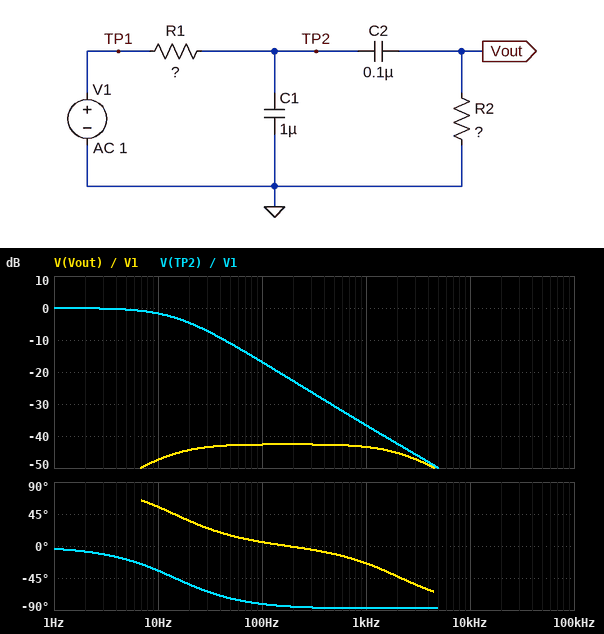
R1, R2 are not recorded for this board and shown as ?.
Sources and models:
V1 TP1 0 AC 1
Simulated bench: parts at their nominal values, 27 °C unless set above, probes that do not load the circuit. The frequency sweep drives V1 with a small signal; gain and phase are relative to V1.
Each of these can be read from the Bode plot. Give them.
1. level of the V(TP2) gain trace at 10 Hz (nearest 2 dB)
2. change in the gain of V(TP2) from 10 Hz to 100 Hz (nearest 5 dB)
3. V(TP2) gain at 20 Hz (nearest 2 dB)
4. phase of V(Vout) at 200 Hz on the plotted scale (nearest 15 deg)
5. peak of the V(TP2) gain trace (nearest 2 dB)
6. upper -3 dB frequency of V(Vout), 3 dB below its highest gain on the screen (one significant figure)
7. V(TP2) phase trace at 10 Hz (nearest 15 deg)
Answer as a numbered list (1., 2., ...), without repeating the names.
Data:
1. -2 dB
2. -15 dB
3. -4 dB
4. 0 deg
5. 0 dB
6. 2 kHz
7. -30 deg
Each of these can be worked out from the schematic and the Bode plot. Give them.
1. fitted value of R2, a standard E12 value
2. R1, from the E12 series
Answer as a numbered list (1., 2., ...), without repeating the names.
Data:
1. 820 Ω
2. 10 kΩ
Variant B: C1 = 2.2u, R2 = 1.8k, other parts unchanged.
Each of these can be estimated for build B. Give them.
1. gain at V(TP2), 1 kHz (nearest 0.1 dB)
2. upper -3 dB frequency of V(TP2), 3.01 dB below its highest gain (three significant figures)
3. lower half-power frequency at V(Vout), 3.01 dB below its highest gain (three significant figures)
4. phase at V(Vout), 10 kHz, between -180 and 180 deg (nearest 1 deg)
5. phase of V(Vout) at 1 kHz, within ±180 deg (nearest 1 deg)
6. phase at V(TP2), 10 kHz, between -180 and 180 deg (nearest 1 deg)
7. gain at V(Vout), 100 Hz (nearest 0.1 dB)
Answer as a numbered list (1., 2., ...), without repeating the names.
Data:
1. -43.0 dB
2. 6.92 Hz
3. 6.82 Hz
4. -85 deg
5. -47 deg
6. -90 deg
7. -42.2 dB
